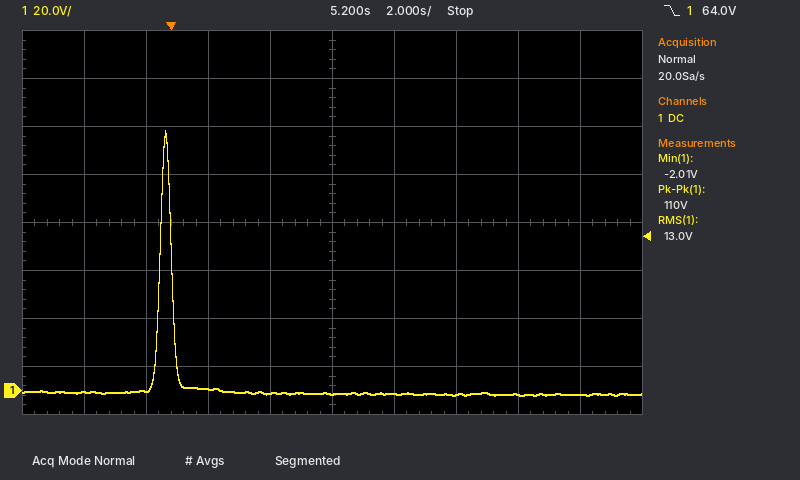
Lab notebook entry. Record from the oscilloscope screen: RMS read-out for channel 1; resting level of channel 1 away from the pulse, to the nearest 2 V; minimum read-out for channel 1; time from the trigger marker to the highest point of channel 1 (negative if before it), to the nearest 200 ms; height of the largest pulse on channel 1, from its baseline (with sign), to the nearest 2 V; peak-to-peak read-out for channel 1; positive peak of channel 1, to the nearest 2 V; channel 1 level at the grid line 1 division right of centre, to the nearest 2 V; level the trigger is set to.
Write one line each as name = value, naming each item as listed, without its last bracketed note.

RMS read-out for channel 1 = 13.0 V
resting level of channel 1 away from the pulse, to the nearest 2 V = -2 V
minimum read-out for channel 1 = -2.01 V
time from the trigger marker to the highest point of channel 1 (negative if before it), to the nearest 200 ms = -200 ms
height of the largest pulse on channel 1, from its baseline (with sign), to the nearest 2 V = +110 V
peak-to-peak read-out for channel 1 = 110 V
positive peak of channel 1, to the nearest 2 V = 108 V
channel 1 level at the grid line 1 division right of centre, to the nearest 2 V = -2 V
level the trigger is set to = 64.0 V
